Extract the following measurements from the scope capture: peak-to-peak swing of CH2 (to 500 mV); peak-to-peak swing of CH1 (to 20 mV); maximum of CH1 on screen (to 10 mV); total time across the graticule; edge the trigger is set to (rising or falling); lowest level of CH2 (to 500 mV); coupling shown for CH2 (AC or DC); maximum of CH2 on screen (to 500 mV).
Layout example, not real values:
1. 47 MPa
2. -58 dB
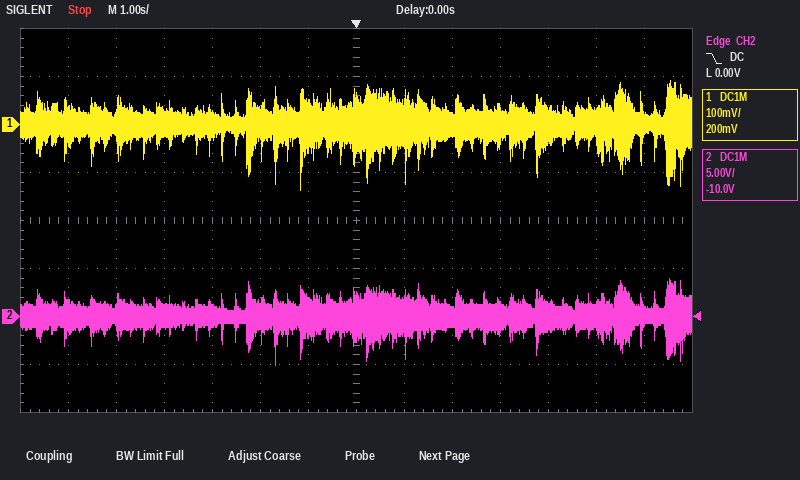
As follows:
1. 9.0 V
2. 220 mV
3. 90 mV
4. 14 s
5. falling
6. -5.0 V
7. DC
8. 4.0 V
